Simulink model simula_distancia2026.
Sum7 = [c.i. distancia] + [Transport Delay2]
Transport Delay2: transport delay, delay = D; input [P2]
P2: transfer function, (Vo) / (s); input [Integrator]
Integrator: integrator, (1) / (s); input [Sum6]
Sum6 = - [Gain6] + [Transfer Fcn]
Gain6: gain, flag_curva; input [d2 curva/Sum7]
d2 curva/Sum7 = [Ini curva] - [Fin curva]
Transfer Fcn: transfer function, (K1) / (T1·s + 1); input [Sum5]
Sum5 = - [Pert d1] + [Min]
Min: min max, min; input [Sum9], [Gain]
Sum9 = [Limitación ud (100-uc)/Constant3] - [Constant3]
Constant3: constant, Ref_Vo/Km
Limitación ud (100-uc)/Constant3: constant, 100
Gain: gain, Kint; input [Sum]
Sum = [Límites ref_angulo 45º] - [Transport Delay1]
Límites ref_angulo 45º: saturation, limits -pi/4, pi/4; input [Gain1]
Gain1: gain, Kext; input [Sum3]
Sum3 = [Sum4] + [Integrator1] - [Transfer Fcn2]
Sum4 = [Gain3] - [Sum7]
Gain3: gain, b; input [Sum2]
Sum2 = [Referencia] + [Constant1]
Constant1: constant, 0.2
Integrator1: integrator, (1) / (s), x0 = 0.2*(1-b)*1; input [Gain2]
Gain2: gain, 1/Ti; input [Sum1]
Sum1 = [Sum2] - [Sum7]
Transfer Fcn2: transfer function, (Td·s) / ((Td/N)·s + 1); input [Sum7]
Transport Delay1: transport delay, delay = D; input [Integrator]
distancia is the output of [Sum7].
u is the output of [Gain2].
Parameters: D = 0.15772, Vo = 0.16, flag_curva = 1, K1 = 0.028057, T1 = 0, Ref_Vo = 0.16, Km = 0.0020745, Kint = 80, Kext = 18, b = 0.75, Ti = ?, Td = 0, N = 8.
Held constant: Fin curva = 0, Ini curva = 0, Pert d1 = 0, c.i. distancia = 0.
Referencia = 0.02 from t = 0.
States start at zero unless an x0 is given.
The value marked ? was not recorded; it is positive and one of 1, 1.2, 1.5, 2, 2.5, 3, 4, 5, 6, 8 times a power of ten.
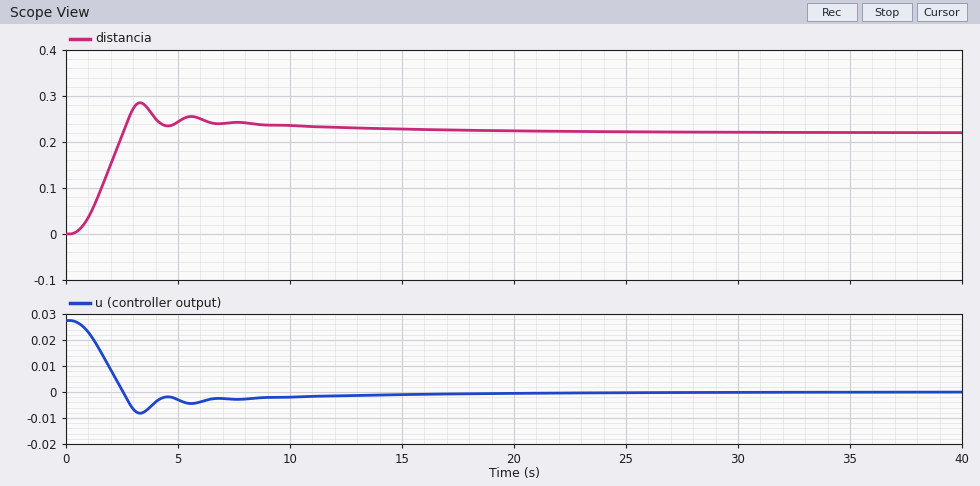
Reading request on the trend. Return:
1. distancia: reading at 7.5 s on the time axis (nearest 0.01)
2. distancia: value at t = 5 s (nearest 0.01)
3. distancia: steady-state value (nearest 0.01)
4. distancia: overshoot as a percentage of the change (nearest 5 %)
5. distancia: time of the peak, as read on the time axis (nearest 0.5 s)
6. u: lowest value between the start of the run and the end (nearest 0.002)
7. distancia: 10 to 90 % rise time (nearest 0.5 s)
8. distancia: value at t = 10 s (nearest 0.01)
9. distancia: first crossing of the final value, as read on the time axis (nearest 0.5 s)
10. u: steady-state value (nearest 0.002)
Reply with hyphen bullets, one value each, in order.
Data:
- 0.24
- 0.24
- 0.22
- 30 %
- 3.5 s
- -0.008
- 1.5 s
- 0.24
- 2.5 s
- 0.000
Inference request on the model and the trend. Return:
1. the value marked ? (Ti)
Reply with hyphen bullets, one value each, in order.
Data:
- 8
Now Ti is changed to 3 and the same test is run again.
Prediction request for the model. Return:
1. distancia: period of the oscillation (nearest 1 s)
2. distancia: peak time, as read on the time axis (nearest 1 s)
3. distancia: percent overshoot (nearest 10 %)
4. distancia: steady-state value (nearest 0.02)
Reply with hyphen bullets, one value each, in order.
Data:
- 3 s
- 4 s
- 60 %
- 0.22
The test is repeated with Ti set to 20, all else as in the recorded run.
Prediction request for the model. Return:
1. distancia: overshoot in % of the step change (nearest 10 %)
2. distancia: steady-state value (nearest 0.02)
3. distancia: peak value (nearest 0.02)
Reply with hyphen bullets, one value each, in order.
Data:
- 20 %
- 0.22
- 0.26
